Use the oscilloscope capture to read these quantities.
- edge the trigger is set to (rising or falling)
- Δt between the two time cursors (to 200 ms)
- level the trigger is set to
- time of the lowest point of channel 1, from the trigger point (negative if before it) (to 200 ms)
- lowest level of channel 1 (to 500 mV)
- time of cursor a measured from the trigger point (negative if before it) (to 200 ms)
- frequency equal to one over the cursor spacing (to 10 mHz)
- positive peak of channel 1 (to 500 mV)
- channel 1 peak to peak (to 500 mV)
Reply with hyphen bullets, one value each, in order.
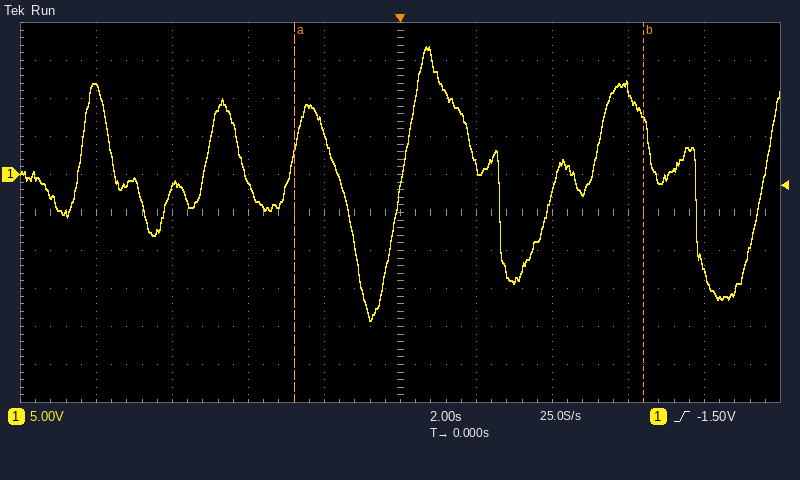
- rising
- 9.2 s
- -1.50 V
- -800 ms
- -19.0 V
- -2.8 s
- 110 mHz
- 17.0 V
- 36.0 V
